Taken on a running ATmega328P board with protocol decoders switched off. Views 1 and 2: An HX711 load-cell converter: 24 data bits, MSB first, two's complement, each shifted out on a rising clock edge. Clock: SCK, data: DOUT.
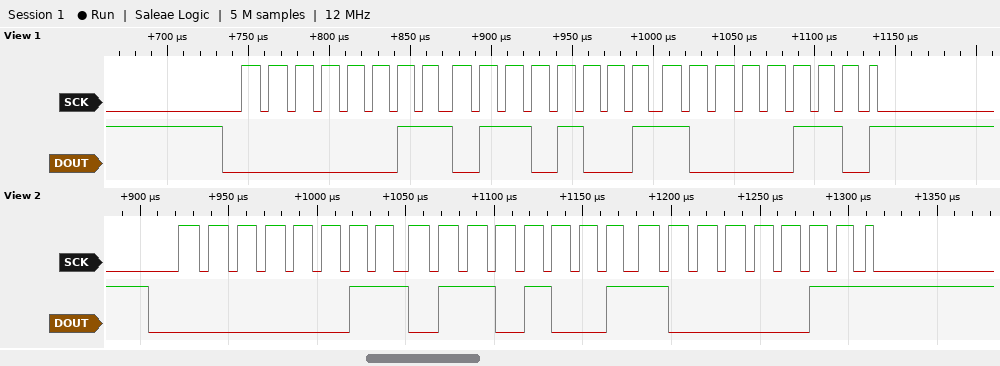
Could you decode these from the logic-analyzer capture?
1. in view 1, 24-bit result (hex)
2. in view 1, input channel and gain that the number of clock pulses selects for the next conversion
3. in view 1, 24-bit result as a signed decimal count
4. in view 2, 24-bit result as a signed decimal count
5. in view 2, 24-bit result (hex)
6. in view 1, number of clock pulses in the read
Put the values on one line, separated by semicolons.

0x036986; channel A, gain 128; 223622; 223619; 0x036983; 25
